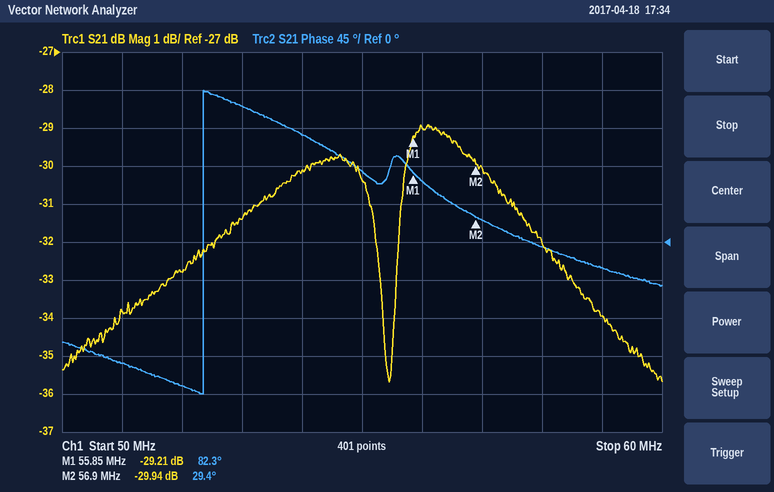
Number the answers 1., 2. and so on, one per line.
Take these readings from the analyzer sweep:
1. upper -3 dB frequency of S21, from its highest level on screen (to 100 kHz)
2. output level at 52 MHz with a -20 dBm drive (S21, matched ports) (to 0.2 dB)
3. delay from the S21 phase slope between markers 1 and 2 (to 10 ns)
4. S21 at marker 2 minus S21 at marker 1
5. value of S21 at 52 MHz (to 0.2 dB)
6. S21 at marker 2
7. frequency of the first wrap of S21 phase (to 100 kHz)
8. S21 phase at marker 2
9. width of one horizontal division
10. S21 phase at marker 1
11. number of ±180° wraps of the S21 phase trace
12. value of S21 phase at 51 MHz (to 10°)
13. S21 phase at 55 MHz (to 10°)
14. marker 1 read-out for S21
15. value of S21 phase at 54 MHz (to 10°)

1. 58.0 MHz
2. -52.8 dBm
3. 140 ns
4. -0.73 dB
5. -32.8 dB
6. -29.94 dB
7. 52.4 MHz
8. 29.4°
9. 1 MHz
10. 82.3°
11. 1
12. -140°
13. 80°
14. -29.21 dB
15. 130°
